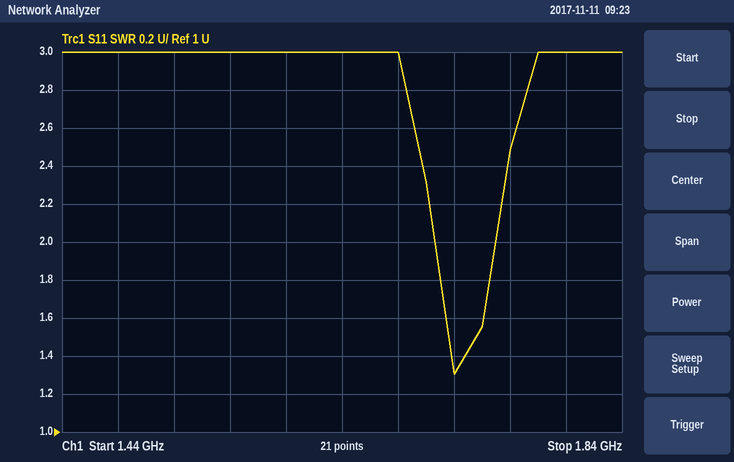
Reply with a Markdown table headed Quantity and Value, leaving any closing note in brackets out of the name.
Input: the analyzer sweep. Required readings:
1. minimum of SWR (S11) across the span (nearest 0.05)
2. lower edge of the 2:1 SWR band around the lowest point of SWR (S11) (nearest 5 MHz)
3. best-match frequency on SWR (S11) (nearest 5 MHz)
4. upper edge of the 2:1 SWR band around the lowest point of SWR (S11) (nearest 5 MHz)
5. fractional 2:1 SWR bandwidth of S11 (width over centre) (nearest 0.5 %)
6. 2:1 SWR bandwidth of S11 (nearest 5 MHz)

| Quantity | Value |
|---|---|
| minimum of SWR (S11) across the span | 1.30 |
| lower edge of the 2:1 SWR band around the lowest point of SWR (S11) | 1.705 GHz |
| best-match frequency on SWR (S11) | 1.720 GHz |
| upper edge of the 2:1 SWR band around the lowest point of SWR (S11) | 1.750 GHz |
| fractional 2:1 SWR bandwidth of S11 (width over centre) | 2.5 % |
| 2:1 SWR bandwidth of S11 | 45 MHz |
